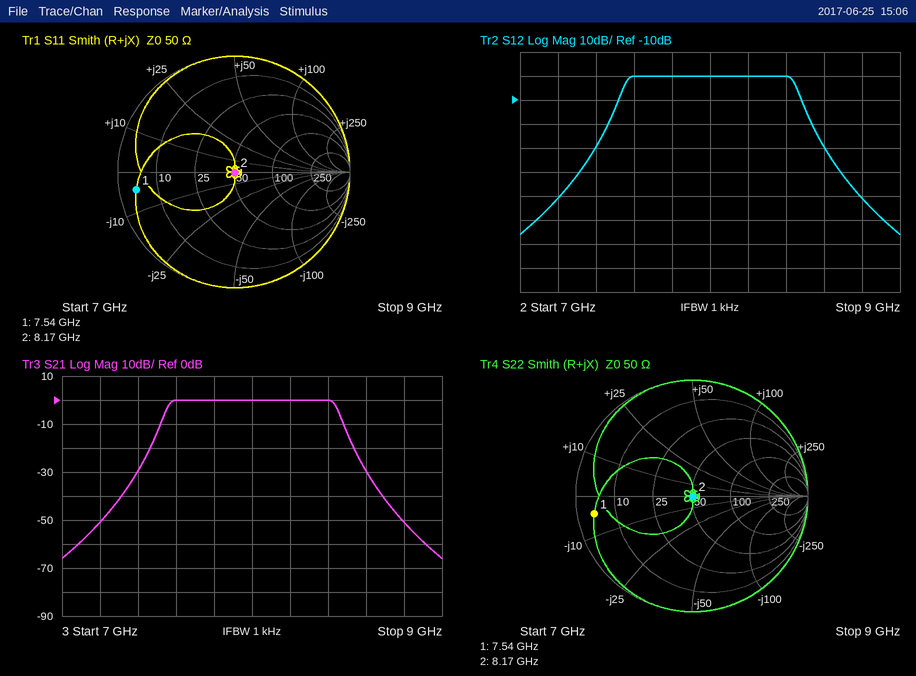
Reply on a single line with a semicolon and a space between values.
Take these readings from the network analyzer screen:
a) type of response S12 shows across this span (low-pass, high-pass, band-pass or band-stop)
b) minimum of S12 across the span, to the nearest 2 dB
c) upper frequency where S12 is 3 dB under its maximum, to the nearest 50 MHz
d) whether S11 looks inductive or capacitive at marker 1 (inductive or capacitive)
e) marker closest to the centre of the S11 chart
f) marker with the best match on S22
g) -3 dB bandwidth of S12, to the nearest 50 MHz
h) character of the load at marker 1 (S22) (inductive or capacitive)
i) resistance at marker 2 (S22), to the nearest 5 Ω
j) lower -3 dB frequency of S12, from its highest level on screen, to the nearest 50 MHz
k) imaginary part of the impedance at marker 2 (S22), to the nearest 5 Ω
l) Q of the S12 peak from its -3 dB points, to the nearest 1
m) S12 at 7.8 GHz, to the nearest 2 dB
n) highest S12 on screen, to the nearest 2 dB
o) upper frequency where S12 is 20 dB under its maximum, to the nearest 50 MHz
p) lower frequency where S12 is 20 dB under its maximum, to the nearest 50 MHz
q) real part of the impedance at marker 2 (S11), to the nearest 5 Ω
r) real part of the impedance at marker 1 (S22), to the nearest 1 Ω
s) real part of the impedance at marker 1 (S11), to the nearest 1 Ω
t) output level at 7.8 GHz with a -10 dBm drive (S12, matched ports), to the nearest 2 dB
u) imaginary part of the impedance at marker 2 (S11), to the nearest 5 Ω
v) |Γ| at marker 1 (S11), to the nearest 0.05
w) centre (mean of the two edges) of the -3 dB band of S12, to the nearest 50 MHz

band-pass; -66 dB; 8.45 GHz; capacitive; marker 2; marker 2; 900 MHz; capacitive; 50 Ω; 7.55 GHz; 0 Ω; 9; 0 dB; 0 dB; 8.55 GHz; 7.45 GHz; 50 Ω; 4 Ω; 4 Ω; -10 dBm; 0 Ω; 0.85; 8.00 GHz
